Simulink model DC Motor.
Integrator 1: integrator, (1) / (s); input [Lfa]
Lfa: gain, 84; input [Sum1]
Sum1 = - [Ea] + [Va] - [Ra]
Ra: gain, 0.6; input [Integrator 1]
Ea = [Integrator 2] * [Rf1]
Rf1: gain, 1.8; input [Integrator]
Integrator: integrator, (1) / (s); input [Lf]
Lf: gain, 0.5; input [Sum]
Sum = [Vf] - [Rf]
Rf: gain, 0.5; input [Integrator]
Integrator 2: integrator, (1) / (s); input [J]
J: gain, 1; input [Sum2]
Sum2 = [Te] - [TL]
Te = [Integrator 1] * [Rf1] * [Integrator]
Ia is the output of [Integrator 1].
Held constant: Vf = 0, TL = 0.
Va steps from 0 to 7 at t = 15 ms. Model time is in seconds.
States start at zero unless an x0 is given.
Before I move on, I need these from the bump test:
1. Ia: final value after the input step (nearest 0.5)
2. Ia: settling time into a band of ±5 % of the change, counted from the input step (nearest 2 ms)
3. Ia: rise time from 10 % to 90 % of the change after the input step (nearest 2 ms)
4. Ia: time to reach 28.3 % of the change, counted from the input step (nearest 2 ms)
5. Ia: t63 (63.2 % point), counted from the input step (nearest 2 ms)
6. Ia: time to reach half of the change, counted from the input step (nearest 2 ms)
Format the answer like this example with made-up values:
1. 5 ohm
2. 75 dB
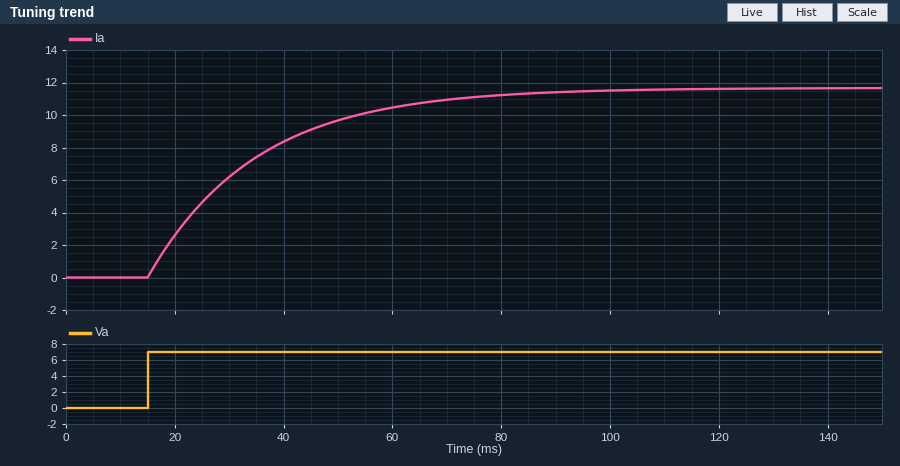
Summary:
1. 11.5
2. 60 ms
3. 44 ms
4. 6 ms
5. 20 ms
6. 14 ms
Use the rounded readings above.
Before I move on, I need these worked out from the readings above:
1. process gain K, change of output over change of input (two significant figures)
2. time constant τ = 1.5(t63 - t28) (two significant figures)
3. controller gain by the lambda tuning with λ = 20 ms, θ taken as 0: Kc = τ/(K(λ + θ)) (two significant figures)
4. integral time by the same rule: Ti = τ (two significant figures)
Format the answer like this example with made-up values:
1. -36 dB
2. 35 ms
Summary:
1. 1.6
2. 21 ms
3. 0.66
4. 21 ms
